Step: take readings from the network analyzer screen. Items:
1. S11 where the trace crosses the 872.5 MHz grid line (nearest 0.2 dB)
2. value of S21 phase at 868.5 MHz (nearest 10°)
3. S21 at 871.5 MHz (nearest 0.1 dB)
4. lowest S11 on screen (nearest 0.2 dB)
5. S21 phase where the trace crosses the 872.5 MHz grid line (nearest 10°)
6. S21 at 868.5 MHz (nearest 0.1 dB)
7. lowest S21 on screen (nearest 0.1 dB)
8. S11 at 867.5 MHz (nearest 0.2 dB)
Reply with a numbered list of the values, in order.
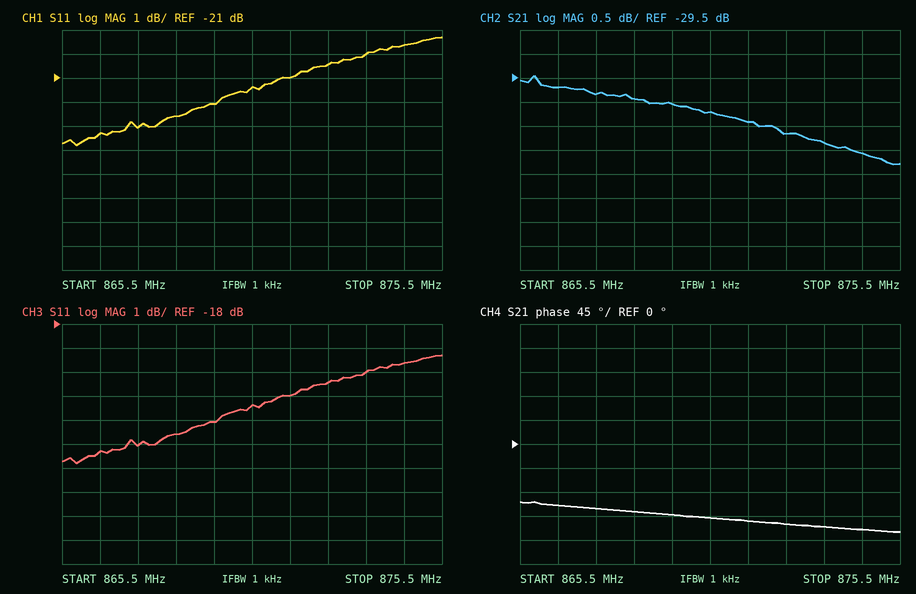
1. -20.4 dB
2. -130°
3. -30.4 dB
4. -23.8 dB
5. -150°
6. -29.9 dB
7. -31.3 dB
8. -23.0 dB
